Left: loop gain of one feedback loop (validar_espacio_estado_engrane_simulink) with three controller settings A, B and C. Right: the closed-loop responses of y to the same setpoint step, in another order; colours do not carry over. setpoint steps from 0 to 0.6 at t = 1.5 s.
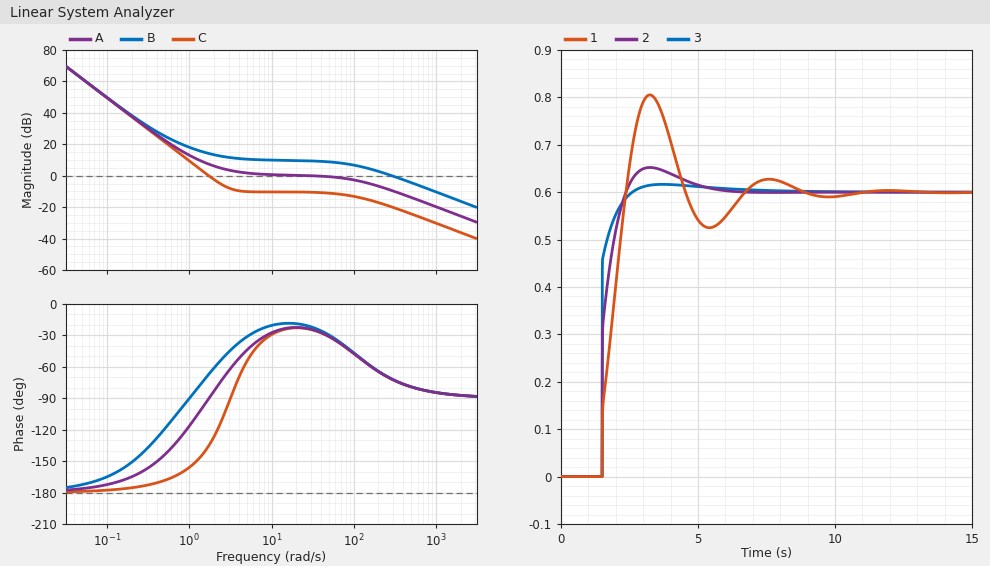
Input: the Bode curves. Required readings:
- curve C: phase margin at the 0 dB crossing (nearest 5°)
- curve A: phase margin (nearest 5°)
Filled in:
45°
155°
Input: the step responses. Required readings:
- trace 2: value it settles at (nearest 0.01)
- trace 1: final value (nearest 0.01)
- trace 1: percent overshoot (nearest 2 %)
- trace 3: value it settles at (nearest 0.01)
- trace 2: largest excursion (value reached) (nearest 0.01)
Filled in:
0.60
0.60
34 %
0.60
0.65
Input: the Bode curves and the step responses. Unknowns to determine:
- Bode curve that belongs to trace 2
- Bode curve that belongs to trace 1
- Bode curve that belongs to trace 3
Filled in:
A
C
B
